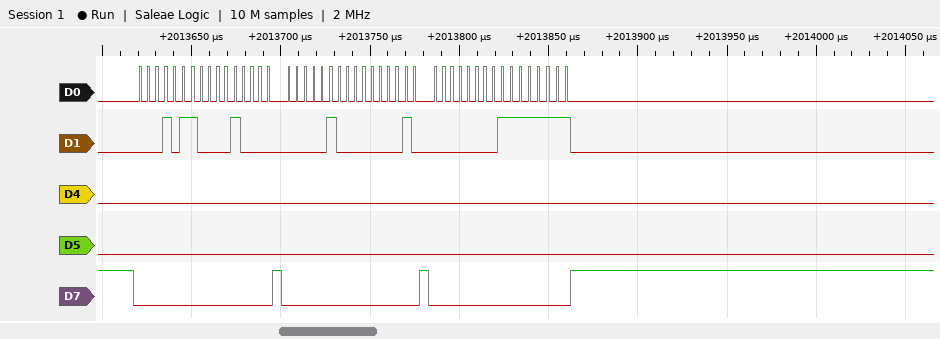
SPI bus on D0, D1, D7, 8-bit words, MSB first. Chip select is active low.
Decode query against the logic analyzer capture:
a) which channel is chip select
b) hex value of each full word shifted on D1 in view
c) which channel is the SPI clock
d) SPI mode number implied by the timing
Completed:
D7
16, 10, 04, 02, 00, FF
D0
1
